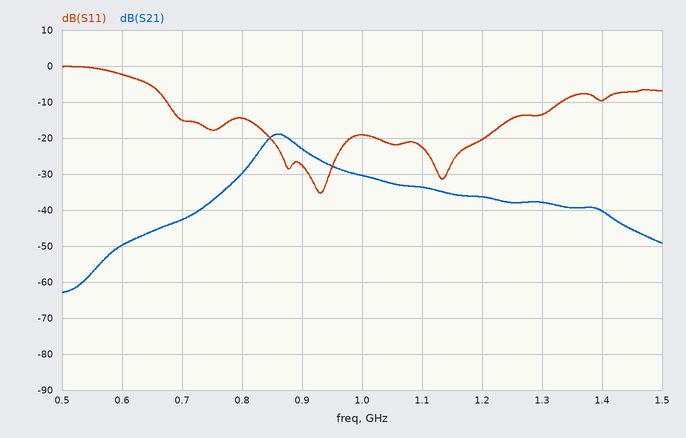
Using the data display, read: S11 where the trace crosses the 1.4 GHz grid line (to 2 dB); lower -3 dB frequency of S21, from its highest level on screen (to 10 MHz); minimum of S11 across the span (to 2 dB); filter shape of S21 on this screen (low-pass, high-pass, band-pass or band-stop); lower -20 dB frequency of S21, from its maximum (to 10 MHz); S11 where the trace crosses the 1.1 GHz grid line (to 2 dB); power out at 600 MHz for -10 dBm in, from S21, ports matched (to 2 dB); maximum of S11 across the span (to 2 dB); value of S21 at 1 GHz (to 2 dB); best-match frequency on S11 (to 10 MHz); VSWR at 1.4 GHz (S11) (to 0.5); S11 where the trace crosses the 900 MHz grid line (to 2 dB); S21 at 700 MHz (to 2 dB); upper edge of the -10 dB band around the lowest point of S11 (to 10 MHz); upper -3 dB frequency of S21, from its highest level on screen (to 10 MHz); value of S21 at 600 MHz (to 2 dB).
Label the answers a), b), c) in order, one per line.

a) -10 dB
b) 840 MHz
c) -36 dB
d) band-pass
e) 740 MHz
f) -22 dB
g) -60 dBm
h) 0 dB
i) -30 dB
j) 930 MHz
k) 2.0
l) -28 dB
m) -42 dB
n) 1.33 GHz
o) 890 MHz
p) -50 dB
